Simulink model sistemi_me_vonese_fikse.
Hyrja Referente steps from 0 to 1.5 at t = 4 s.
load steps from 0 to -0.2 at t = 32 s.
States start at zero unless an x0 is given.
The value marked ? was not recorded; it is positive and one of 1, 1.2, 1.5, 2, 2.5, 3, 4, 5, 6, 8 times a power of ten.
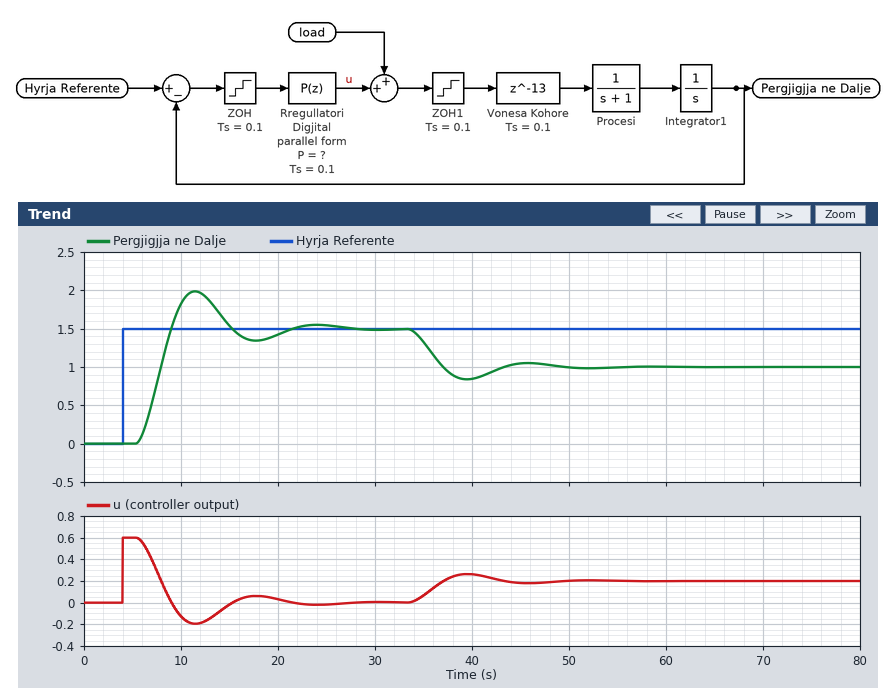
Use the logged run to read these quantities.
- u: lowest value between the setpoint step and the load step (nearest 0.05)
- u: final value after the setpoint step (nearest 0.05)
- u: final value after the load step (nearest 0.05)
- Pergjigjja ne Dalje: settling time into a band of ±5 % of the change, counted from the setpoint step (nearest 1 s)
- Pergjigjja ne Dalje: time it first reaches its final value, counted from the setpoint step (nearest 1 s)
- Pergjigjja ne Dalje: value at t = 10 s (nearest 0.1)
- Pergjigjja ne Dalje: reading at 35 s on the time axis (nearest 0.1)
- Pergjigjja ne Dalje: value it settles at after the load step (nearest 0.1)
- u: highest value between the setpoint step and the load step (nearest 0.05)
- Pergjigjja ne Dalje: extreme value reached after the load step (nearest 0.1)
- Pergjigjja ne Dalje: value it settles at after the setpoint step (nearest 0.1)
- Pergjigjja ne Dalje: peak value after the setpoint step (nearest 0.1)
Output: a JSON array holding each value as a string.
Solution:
["-0.20", "0.00", "0.20", "16 s", "5 s", "1.8", "1.3", "1.0", "0.60", "0.8", "1.5", "2.0"]
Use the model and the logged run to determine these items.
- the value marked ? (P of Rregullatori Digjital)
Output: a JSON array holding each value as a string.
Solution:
["0.4"]
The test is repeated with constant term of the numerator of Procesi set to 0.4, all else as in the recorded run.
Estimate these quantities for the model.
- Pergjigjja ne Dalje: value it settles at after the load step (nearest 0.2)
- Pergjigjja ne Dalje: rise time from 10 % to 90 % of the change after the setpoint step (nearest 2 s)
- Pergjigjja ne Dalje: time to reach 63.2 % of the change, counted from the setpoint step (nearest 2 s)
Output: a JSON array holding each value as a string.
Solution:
["1.0", "8 s", "6 s"]
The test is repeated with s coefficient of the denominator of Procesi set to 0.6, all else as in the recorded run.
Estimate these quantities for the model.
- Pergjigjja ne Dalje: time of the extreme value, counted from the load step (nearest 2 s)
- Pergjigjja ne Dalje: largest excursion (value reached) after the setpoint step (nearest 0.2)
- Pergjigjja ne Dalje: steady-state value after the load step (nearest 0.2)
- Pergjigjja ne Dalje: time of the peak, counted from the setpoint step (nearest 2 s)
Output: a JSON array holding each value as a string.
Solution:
["6 s", "1.8", "1.0", "6 s"]
